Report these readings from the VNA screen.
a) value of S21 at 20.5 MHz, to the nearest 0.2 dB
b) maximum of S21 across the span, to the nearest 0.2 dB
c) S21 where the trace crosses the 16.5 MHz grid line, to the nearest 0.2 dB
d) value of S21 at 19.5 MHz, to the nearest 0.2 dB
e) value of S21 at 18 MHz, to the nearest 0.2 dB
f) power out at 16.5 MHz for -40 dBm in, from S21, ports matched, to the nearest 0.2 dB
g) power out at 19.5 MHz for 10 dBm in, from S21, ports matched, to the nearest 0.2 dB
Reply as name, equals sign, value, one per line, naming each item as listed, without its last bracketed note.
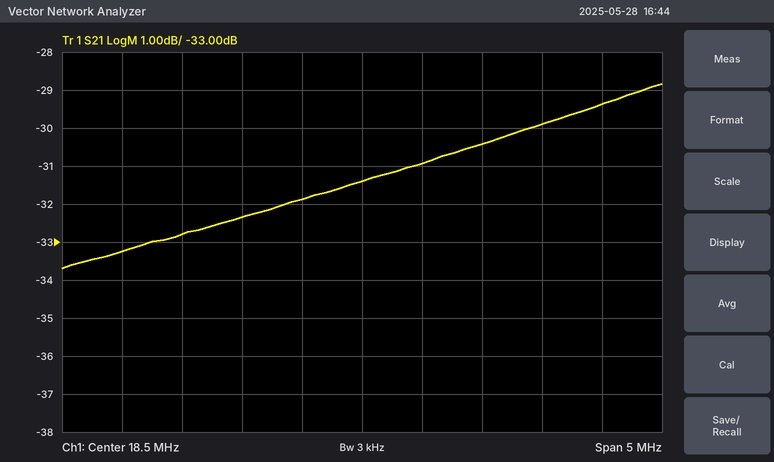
value of S21 at 20.5 MHz, to the nearest 0.2 dB = -29.4 dB
maximum of S21 across the span, to the nearest 0.2 dB = -28.8 dB
S21 where the trace crosses the 16.5 MHz grid line, to the nearest 0.2 dB = -33.2 dB
value of S21 at 19.5 MHz, to the nearest 0.2 dB = -30.4 dB
value of S21 at 18 MHz, to the nearest 0.2 dB = -31.8 dB
power out at 16.5 MHz for -40 dBm in, from S21, ports matched, to the nearest 0.2 dB = -73.2 dBm
power out at 19.5 MHz for 10 dBm in, from S21, ports matched, to the nearest 0.2 dB = -20.4 dBm
